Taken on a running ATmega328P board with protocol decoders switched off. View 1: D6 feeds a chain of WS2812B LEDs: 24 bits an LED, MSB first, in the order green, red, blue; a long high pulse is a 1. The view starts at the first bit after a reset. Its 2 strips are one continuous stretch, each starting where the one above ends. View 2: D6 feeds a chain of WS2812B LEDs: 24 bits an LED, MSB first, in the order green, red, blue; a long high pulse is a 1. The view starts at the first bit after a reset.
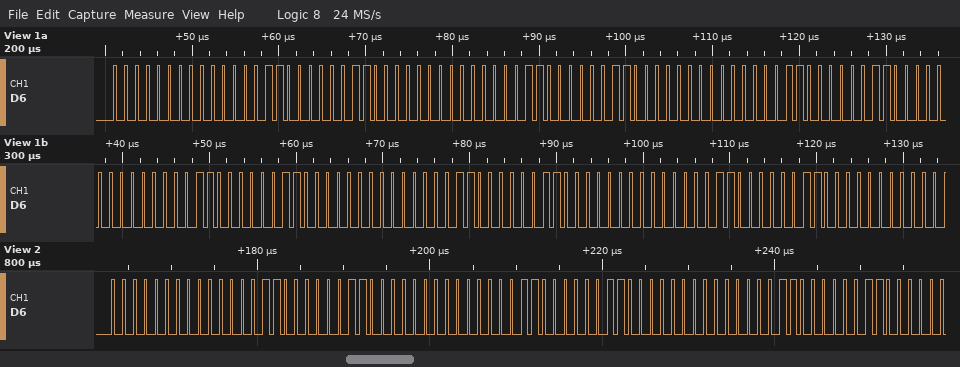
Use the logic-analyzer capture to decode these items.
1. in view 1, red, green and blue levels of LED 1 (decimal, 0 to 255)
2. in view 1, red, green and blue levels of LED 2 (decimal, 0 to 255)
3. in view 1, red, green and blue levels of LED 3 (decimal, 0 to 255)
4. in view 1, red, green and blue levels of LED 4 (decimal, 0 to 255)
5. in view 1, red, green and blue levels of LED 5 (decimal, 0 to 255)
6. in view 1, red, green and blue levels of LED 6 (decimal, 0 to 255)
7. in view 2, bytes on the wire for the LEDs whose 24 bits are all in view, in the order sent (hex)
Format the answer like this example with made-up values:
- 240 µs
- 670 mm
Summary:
- 3, 0, 3
- 3, 0, 3
- 3, 0, 3
- 3, 0, 3
- 3, 0, 3
- 3, 0, 3
- 00 03 03 00 03 03 00 03 03
